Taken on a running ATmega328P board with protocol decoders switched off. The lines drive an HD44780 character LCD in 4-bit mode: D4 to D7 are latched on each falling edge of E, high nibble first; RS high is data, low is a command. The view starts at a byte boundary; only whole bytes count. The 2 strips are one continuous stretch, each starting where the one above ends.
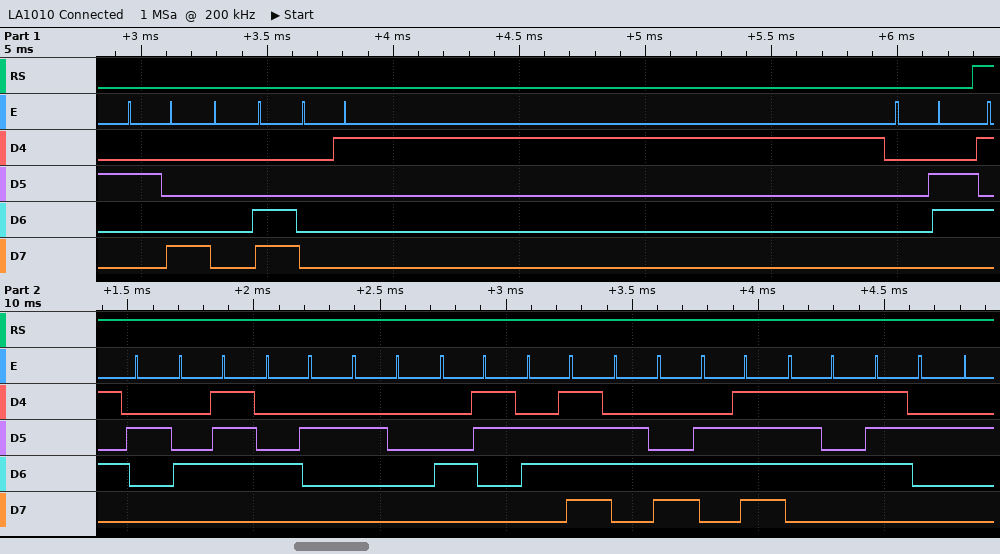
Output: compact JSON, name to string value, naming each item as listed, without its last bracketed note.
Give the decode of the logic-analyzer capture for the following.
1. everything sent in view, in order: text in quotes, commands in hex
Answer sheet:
{"everything sent in view, in order: text in quotes, commands in hex": "0x28 0x0C 0x01 0x06 \"RGB Colour\""}
